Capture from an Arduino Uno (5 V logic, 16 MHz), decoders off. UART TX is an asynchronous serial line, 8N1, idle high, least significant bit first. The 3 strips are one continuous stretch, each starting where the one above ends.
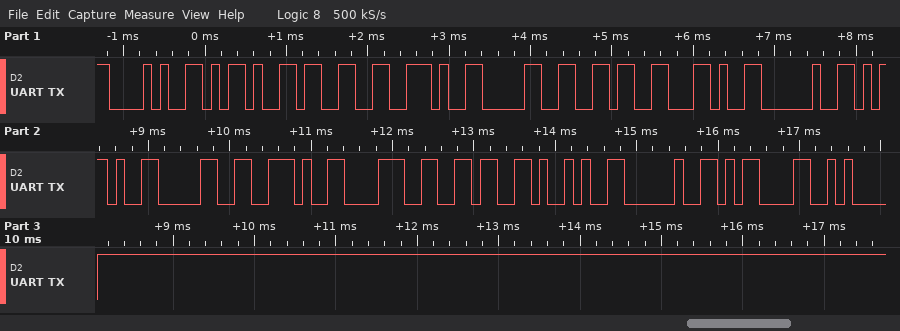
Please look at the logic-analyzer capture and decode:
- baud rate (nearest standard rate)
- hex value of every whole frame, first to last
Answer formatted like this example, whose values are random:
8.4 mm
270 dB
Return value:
9600 baud
0x28 0x2D 0x33 0x2E 0x30 0x36 0x2C 0x20 0x2D 0x30 0x2E 0x38 0x36 0x29 0x20 0x0D 0x0A
